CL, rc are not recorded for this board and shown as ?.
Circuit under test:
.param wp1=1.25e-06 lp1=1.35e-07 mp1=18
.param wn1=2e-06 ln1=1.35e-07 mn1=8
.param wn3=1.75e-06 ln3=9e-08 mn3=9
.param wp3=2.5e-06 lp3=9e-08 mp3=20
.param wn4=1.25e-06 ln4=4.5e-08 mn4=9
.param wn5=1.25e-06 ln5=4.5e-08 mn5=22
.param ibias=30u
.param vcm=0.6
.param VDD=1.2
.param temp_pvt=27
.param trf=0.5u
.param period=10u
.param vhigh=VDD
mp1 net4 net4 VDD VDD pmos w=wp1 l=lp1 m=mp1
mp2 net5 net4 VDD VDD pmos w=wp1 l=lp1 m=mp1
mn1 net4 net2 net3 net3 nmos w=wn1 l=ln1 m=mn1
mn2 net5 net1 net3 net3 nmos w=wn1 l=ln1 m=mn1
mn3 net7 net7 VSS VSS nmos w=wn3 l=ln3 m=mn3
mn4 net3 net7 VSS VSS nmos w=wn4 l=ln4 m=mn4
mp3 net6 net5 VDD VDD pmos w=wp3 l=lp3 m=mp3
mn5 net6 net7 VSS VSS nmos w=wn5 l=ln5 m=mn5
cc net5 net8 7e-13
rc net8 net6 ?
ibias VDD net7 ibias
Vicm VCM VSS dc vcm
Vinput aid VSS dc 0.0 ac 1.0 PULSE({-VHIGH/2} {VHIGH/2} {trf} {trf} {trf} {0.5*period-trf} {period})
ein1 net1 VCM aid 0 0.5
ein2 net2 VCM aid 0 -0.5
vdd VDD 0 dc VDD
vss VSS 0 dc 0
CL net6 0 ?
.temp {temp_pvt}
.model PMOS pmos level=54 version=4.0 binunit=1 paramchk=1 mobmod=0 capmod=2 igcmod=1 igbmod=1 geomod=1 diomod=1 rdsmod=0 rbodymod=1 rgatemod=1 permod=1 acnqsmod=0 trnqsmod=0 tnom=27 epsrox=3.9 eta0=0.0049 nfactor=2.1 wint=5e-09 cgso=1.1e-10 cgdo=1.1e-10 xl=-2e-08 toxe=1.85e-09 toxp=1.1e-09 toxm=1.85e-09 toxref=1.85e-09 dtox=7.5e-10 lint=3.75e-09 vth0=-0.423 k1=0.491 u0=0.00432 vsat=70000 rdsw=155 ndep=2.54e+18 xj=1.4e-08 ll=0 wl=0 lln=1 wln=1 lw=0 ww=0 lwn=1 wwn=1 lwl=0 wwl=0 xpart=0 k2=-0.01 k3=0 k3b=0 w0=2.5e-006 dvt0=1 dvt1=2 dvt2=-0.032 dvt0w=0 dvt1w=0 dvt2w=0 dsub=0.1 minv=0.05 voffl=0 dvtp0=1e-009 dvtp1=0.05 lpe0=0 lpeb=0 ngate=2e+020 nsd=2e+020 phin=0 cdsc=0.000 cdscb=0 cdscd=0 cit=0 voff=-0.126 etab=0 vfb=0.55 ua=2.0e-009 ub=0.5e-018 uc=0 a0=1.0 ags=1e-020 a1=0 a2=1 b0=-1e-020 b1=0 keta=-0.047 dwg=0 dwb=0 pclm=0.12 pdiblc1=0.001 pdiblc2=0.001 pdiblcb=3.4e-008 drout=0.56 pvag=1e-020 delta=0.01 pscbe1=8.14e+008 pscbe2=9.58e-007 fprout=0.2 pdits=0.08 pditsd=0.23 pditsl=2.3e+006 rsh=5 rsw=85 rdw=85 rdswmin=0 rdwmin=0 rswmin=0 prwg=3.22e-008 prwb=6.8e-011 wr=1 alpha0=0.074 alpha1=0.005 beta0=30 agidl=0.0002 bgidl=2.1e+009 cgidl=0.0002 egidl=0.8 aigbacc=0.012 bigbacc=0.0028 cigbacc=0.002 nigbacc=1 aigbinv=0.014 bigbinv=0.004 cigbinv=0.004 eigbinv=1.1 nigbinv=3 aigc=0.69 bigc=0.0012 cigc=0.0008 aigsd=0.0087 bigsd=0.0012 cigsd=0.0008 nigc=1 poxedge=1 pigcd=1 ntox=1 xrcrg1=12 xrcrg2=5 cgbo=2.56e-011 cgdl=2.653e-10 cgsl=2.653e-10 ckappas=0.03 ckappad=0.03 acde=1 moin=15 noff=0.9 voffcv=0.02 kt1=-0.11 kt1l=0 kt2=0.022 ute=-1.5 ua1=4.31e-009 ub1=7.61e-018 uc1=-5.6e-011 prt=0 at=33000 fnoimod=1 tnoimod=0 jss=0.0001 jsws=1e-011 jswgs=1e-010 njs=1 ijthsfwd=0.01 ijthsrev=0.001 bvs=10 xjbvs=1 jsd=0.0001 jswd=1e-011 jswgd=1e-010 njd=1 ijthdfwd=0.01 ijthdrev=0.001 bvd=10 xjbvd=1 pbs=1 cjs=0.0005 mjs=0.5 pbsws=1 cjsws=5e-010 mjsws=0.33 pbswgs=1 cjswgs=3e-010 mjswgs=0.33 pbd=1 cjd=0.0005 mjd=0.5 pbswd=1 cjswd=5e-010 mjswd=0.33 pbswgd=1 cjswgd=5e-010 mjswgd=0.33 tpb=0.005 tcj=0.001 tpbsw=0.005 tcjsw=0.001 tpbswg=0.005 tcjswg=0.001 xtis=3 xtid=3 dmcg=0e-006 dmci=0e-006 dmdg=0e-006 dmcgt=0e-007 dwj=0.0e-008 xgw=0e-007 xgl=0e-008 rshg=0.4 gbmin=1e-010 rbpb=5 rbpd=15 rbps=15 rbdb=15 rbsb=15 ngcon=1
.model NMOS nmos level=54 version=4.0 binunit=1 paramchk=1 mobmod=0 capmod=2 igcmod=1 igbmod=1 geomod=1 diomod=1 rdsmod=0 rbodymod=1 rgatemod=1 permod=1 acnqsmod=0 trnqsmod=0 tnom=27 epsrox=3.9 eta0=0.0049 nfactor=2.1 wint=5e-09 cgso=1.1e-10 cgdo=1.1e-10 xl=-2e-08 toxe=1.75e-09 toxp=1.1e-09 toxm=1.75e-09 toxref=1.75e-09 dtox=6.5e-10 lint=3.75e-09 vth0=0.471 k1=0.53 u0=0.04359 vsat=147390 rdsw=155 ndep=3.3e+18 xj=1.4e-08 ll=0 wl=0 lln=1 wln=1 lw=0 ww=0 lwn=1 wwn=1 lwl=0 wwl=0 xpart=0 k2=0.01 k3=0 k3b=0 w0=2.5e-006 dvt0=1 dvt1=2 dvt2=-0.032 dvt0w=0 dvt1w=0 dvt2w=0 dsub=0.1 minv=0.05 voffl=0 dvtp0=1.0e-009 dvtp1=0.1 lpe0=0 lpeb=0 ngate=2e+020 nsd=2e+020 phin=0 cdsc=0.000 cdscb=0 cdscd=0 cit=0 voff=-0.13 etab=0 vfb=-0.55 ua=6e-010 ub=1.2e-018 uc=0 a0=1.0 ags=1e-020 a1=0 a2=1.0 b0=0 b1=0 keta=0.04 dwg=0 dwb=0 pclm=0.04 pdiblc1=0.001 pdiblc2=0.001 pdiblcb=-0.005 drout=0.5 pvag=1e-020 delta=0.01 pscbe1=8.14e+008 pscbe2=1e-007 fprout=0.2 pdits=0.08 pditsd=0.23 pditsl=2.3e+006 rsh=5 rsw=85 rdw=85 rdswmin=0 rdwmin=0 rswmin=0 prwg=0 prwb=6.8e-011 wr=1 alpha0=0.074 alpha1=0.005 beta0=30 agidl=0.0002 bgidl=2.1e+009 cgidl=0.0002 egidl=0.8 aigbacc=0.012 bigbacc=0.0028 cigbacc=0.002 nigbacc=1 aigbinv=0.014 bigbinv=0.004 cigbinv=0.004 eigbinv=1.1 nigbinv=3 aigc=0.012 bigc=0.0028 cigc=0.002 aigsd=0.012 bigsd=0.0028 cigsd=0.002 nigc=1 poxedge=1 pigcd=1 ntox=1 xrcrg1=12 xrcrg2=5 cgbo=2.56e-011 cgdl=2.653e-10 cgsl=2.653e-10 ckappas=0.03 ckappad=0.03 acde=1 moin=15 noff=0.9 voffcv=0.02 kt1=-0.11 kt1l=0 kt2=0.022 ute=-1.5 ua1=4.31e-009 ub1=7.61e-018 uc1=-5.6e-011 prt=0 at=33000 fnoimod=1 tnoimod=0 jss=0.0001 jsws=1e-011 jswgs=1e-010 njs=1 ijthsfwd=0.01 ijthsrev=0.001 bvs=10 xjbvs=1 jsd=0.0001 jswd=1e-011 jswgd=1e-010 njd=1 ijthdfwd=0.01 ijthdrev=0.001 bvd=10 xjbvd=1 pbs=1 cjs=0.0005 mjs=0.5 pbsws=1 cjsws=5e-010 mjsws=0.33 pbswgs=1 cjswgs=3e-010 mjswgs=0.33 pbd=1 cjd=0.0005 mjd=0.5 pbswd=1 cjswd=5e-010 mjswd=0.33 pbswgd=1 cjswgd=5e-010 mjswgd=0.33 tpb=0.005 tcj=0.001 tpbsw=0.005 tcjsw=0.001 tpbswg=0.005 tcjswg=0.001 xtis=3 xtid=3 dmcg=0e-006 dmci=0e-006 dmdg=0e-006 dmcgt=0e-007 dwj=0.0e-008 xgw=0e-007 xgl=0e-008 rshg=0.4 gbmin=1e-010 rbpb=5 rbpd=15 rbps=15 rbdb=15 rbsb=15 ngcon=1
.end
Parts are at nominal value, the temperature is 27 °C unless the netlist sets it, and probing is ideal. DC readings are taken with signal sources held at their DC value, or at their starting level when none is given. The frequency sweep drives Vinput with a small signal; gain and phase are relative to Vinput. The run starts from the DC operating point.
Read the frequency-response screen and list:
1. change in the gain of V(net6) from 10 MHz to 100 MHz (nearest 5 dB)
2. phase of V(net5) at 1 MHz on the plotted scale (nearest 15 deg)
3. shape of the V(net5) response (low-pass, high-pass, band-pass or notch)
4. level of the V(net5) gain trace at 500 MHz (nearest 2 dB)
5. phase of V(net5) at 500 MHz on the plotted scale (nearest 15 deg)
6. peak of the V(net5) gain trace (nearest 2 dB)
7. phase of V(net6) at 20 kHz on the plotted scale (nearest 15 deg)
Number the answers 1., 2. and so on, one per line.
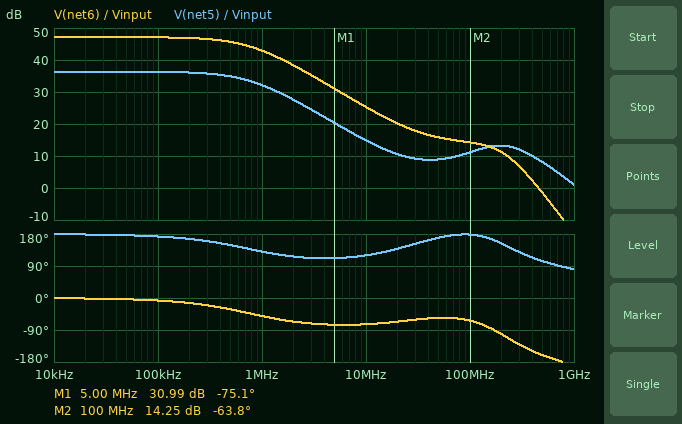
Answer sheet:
1. -10 dB
2. 135 deg
3. low-pass
4. 8 dB
5. 105 deg
6. 36 dB
7. 0 deg
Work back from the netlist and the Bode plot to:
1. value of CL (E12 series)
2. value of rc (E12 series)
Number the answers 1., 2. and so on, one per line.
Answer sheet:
1. 3.3 pF
2. 6.8 kΩ
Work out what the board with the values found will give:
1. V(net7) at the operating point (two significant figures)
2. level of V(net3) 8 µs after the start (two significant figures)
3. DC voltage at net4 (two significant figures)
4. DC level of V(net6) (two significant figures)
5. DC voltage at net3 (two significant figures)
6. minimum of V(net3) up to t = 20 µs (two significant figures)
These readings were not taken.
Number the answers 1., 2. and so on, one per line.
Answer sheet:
1. 360 mV
2. 390 mV
3. 690 mV
4. 170 mV
5. 170 mV
6. 4.3 mV
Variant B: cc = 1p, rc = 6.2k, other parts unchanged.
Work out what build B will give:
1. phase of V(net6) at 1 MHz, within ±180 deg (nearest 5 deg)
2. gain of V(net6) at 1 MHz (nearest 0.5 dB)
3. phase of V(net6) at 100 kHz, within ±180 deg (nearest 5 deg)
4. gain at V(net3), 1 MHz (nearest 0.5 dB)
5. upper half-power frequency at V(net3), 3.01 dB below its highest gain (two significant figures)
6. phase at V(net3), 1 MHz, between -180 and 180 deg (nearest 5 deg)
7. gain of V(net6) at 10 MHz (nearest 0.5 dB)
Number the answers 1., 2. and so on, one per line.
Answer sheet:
1. -60 deg
2. 41.0 dB
3. -10 deg
4. -19.5 dB
5. 560 kHz
6. 130 deg
7. 22.5 dB
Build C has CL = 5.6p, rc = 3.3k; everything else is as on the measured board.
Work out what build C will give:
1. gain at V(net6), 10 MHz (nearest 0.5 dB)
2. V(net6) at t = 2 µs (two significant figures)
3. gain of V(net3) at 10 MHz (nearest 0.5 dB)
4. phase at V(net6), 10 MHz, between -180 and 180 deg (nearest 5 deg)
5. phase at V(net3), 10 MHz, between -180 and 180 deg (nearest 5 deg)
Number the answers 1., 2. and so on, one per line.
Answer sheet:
1. 25.0 dB
2. 1.0 V
3. -30.5 dB
4. -85 deg
5. 150 deg
